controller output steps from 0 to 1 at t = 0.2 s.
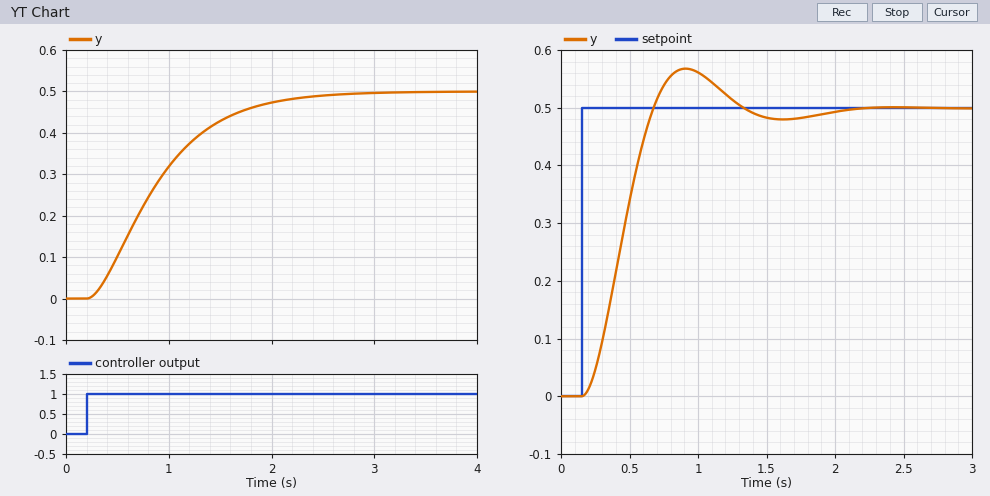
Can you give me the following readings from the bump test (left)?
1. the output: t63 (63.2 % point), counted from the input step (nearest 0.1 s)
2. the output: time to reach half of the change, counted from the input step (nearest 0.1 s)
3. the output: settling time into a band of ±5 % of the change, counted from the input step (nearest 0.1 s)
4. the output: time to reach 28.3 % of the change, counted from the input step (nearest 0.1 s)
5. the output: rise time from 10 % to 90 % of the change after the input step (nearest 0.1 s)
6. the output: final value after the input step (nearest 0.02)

0.8 s
0.6 s
1.8 s
0.4 s
1.3 s
0.50
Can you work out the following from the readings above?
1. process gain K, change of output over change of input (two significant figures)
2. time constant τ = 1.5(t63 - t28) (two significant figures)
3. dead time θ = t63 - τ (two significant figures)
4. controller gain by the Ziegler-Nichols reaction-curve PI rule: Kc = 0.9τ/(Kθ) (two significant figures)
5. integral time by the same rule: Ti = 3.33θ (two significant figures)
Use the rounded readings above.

0.50
0.60 s
0.20 s
5.4
0.67 s
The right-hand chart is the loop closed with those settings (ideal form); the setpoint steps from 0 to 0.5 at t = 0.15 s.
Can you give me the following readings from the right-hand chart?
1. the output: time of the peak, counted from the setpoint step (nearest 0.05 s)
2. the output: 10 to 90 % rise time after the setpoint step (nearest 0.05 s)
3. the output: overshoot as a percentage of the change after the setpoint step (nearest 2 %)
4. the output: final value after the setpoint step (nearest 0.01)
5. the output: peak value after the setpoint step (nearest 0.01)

0.75 s
0.35 s
14 %
0.50
0.57
